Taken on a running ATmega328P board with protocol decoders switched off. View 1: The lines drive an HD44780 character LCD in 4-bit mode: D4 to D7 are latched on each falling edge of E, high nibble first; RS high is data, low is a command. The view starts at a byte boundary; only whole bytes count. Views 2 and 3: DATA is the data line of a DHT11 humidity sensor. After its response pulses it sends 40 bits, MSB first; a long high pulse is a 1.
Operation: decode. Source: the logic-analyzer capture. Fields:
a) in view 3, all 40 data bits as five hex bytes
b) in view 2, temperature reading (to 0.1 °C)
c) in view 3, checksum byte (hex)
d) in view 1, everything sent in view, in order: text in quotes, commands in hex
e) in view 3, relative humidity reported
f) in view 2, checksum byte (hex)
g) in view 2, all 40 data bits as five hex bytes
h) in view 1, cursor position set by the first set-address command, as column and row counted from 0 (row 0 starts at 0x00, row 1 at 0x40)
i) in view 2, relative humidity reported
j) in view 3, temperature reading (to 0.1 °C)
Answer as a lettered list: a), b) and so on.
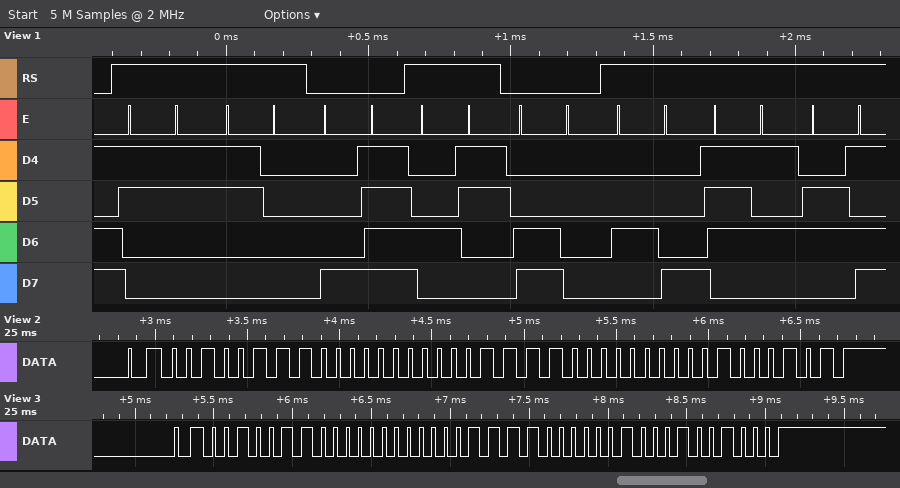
a) 26 00 1E 04 48
b) 30.0 °C
c) 0x48
d) "30" 0x8F "C" 0xC0 "Hum"
e) 38 %
f) 0x45
g) 27 00 1E 00 45
h) column 15, row 0
i) 39 %
j) 30.4 °C
